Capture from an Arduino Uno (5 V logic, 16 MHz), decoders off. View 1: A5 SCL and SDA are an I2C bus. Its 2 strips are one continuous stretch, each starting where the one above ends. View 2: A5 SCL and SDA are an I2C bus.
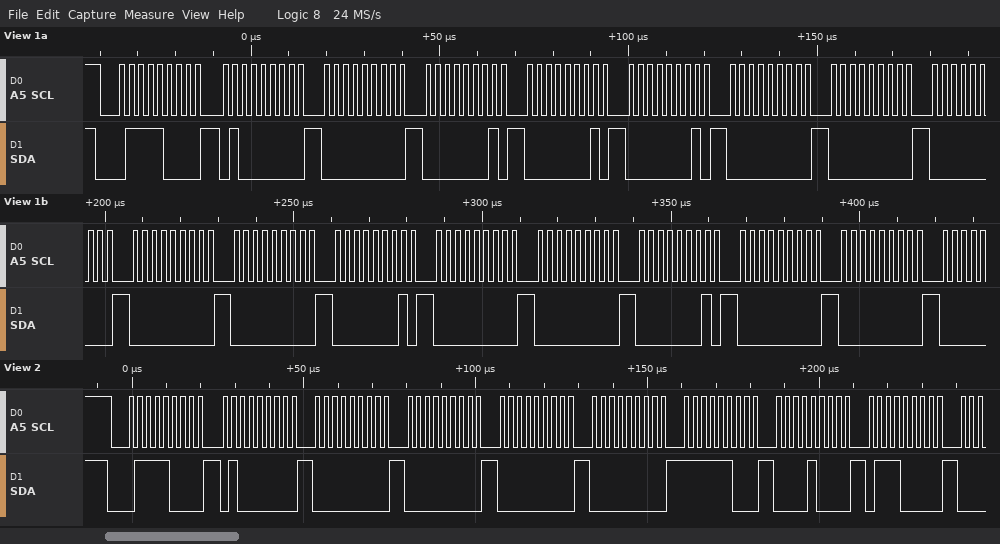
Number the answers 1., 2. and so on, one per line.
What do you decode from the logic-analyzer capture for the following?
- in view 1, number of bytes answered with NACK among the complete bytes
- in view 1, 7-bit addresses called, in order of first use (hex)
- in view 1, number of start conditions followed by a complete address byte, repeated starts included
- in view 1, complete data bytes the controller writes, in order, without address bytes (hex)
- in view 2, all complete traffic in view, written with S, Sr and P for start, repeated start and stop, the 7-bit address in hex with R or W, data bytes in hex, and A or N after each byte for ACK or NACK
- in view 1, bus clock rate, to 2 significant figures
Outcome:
1. 0
2. 0x3C
3. 1
4. 40 00 01 01 01 00 00 00 00 00 01 00 00 01 00 00
5. S 3CW A 40 A 00 A 00 A 00 A 00 A FC A 08 A 70 A
6. 400 kHz
